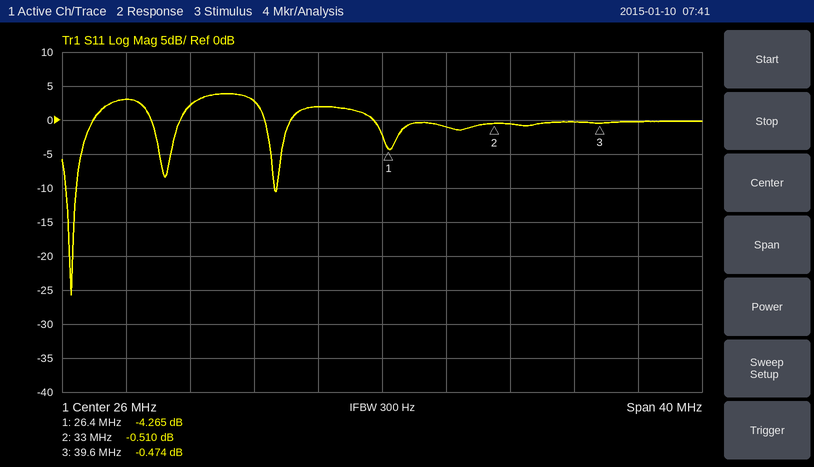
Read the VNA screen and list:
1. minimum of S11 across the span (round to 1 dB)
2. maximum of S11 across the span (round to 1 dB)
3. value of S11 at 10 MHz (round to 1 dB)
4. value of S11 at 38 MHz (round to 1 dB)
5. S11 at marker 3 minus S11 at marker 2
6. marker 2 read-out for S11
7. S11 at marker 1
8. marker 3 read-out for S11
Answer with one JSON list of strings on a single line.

["-26 dB", "4 dB", "3 dB", "0 dB", "0.036 dB", "-0.510 dB", "-4.265 dB", "-0.474 dB"]
